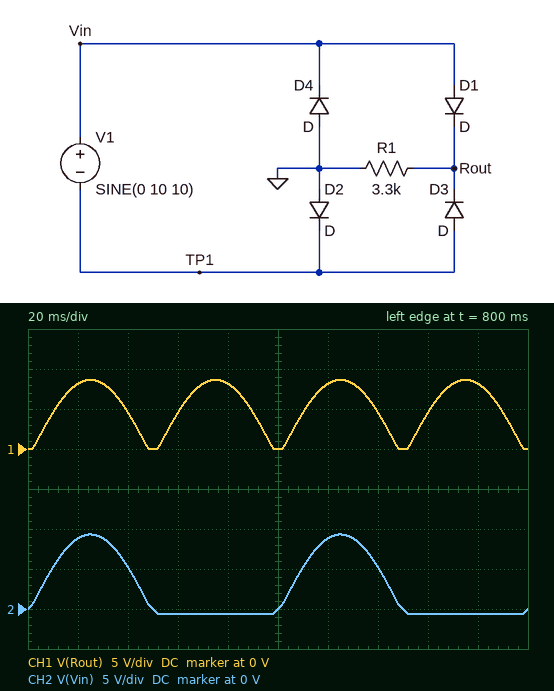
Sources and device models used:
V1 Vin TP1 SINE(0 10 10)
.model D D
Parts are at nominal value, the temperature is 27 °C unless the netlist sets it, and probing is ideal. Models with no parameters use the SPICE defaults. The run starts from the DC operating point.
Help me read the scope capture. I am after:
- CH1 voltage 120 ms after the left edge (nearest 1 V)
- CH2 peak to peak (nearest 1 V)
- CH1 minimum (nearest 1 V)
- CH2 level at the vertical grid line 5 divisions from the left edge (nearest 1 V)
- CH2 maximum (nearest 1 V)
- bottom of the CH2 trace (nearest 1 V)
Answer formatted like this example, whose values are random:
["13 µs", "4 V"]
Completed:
["8 V", "10 V", "0 V", "0 V", "9 V", "-1 V"]
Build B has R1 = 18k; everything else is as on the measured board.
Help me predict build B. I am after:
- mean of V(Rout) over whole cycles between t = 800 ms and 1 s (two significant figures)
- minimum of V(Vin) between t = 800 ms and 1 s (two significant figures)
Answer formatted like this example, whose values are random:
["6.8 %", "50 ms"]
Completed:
["5.2 V", "-640 mV"]
